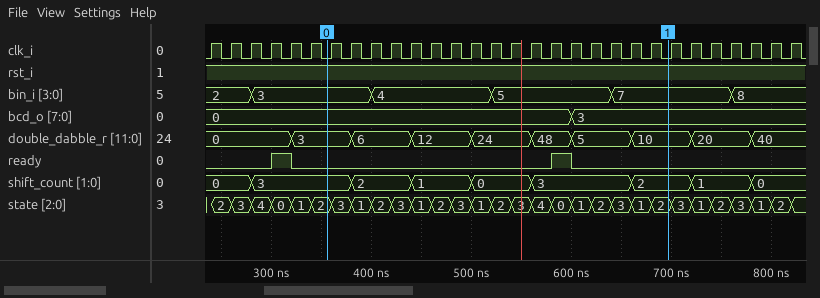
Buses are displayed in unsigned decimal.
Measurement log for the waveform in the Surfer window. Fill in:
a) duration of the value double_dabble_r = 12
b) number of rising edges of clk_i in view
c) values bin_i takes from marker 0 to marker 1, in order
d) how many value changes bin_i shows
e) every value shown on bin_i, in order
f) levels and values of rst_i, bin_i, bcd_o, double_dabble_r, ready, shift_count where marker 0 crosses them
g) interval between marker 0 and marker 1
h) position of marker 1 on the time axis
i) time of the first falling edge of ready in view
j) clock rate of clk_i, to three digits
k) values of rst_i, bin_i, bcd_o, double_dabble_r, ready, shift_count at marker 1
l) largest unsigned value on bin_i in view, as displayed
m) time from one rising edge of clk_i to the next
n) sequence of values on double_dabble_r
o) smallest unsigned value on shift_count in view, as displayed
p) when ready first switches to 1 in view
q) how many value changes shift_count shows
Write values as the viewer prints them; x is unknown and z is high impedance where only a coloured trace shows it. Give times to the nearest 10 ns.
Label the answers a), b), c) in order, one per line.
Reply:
a) 60 ns
b) 30
c) 3, 4, 5, 7
d) 5
e) 2, 3, 4, 5, 7, 8
f) rst_i=1, bin_i=3, bcd_o=0, double_dabble_r=3, ready=0, shift_count=3
g) 340 ns
h) 700 ns
i) 320 ns
j) 50.0 MHz
k) rst_i=1, bin_i=7, bcd_o=3, double_dabble_r=10, ready=0, shift_count=2
l) 8
m) 20 ns
n) 0, 3, 6, 12, 24, 48, 5, 10, 20, 40
o) 0
p) 300 ns
q) 8
